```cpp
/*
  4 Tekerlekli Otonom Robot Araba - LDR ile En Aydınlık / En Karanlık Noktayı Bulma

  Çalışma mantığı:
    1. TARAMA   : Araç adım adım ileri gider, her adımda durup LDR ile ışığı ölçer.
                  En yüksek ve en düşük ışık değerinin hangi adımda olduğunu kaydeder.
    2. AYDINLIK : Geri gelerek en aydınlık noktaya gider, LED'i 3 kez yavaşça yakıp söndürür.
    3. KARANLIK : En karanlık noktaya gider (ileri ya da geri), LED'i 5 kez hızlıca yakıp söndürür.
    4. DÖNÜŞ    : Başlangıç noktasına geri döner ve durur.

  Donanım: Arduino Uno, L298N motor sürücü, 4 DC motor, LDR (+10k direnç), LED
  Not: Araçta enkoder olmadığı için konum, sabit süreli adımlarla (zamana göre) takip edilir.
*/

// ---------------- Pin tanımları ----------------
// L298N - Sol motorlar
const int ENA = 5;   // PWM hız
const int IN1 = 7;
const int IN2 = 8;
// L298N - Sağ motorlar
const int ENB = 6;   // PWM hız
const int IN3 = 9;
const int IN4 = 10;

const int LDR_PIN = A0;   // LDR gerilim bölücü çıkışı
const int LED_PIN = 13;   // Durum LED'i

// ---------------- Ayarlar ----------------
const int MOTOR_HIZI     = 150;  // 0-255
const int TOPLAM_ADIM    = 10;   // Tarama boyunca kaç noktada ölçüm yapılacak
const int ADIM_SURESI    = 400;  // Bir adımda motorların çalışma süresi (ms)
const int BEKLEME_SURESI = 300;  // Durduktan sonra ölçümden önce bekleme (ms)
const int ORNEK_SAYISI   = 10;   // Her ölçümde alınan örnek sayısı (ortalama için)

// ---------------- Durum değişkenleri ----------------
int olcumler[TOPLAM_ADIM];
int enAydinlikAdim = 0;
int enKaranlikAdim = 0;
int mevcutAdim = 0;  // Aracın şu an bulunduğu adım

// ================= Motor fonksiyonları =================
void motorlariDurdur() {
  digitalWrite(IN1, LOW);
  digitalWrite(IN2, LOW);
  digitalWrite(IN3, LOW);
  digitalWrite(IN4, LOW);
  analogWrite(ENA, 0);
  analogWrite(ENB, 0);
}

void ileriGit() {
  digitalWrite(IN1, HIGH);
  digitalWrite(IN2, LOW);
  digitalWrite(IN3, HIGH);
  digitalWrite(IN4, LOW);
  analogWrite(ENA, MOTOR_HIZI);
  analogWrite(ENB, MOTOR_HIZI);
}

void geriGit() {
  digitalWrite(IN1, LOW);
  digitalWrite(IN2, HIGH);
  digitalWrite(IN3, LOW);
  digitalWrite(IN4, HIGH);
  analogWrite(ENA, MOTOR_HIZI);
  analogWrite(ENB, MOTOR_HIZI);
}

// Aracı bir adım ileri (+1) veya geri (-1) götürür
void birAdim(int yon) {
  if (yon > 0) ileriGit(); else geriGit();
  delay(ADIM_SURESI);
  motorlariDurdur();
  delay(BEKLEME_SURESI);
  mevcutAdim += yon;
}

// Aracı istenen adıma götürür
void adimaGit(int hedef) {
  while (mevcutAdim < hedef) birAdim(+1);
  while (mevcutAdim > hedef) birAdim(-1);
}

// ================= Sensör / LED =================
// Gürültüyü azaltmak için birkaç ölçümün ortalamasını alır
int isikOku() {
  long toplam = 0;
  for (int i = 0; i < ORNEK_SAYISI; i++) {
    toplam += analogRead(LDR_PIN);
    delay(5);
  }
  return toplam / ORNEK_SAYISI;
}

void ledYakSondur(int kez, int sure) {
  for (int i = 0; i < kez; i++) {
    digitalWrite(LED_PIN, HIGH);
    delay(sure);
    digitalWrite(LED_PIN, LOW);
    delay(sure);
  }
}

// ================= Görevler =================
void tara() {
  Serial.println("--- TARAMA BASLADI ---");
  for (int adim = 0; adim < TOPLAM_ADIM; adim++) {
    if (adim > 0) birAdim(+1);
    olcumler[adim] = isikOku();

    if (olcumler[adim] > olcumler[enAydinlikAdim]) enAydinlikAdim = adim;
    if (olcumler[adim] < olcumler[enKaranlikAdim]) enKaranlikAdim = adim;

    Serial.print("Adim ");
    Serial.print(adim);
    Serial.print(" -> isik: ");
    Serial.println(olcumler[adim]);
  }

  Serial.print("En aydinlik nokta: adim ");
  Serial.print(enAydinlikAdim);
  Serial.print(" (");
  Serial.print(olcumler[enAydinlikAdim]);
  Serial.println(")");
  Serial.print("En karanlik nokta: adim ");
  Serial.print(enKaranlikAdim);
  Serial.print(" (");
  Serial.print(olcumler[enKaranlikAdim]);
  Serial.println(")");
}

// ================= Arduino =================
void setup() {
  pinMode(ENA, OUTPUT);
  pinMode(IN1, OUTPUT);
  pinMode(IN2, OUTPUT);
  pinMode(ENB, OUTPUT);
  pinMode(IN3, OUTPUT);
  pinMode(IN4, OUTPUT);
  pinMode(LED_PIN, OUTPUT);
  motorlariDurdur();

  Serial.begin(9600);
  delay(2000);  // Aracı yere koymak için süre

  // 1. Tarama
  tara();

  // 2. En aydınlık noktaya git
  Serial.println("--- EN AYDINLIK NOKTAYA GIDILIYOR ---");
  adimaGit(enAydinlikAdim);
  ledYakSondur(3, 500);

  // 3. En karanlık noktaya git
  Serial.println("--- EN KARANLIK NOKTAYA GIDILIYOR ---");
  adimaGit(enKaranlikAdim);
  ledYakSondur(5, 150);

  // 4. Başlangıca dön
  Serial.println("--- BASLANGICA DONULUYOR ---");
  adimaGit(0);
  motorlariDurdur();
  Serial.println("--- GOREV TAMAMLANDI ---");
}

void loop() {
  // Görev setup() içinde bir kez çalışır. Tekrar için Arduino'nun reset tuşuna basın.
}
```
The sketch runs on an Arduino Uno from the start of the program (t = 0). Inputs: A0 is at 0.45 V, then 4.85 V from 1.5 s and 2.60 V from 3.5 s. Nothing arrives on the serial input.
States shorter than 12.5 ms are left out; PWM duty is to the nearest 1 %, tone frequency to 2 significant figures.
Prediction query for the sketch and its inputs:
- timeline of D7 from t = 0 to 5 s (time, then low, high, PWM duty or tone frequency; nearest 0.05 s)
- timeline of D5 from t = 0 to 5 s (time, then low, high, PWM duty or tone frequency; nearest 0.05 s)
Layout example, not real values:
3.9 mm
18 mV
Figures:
0 s low; 2.05 s high; 2.45 s low; 2.8 s high; 3.2 s low; 3.55 s high; 3.95 s low; 4.3 s high; 4.7 s low
0 s low; 2.05 s PWM 59 %; 2.45 s low; 2.8 s PWM 59 %; 3.2 s low; 3.55 s PWM 59 %; 3.95 s low; 4.3 s PWM 59 %; 4.7 s low
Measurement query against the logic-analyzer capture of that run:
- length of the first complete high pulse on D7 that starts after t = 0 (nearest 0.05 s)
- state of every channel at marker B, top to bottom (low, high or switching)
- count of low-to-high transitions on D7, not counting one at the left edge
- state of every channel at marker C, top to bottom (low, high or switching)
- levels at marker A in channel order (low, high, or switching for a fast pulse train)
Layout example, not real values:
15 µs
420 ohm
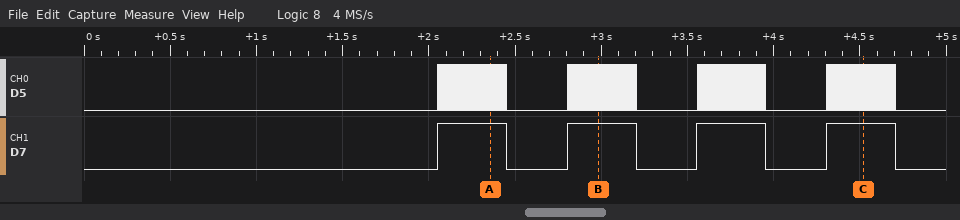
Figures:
0.40 s
D5 switching, D7 high
4
D5 switching, D7 high
D5 switching, D7 high
